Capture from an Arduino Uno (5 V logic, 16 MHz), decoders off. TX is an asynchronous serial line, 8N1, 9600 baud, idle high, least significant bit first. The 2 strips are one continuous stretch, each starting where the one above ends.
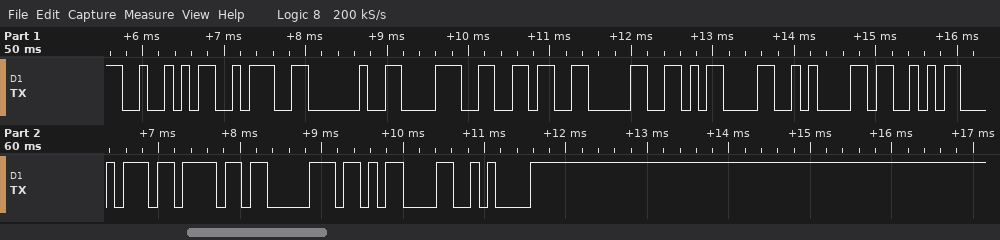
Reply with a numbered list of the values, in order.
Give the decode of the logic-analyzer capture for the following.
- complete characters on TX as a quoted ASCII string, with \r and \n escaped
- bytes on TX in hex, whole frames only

1. "R: 860\r\nStop\r\n"
2. 52 3A 20 38 36 30 0D 0A 53 74 6F 70 0D 0A
